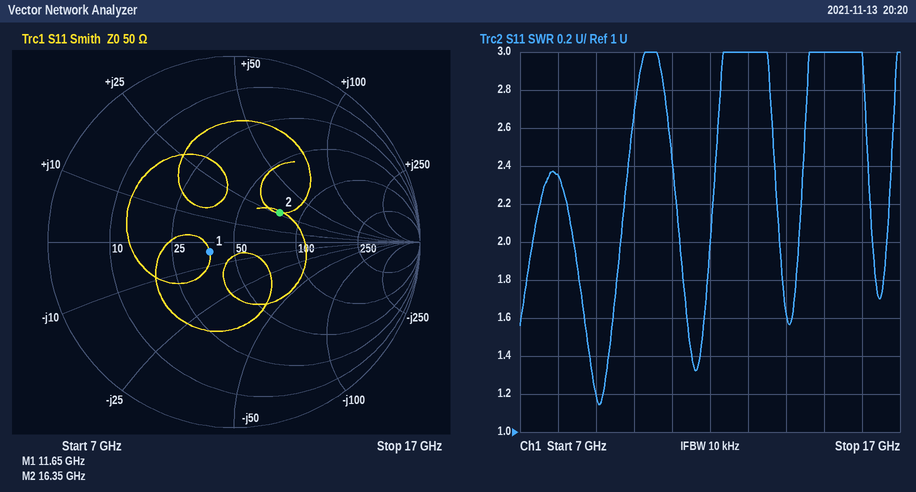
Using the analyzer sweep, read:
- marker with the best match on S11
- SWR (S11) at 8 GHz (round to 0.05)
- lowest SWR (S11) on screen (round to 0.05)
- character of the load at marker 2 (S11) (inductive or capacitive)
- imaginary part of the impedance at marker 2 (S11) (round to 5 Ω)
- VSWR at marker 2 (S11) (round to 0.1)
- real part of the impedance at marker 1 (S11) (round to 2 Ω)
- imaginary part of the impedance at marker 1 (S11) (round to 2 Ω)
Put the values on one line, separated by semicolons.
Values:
marker 1; 2.35; 1.15; inductive; +25 Ω; 1.8; 38 Ω; -4 Ω
